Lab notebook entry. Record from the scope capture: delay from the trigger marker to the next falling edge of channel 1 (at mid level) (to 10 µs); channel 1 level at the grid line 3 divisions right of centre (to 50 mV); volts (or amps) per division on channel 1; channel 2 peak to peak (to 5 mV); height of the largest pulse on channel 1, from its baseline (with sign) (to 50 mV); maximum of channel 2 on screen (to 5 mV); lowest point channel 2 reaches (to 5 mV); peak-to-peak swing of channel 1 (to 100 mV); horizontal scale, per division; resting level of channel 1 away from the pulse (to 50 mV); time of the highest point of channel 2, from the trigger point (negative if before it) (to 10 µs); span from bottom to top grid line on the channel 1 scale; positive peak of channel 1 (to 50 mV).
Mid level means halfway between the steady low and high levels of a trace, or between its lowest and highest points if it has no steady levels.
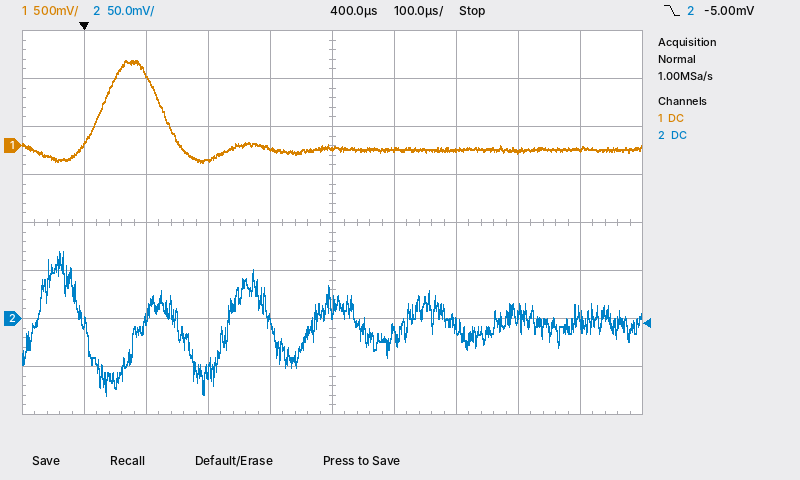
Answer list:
130 µs
-50 mV
500 mV
150 mV
+950 mV
70 mV
-80 mV
1.10 V
100 µs
-50 mV
-40 µs
4 V
900 mV
